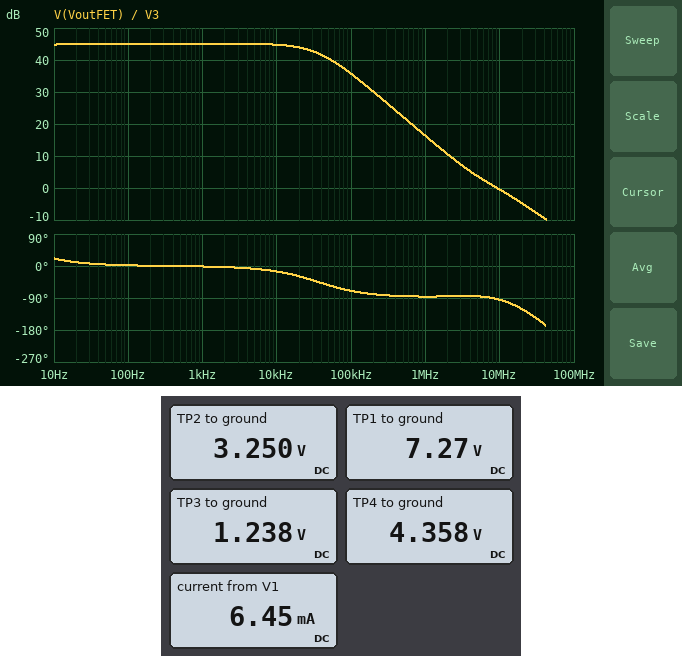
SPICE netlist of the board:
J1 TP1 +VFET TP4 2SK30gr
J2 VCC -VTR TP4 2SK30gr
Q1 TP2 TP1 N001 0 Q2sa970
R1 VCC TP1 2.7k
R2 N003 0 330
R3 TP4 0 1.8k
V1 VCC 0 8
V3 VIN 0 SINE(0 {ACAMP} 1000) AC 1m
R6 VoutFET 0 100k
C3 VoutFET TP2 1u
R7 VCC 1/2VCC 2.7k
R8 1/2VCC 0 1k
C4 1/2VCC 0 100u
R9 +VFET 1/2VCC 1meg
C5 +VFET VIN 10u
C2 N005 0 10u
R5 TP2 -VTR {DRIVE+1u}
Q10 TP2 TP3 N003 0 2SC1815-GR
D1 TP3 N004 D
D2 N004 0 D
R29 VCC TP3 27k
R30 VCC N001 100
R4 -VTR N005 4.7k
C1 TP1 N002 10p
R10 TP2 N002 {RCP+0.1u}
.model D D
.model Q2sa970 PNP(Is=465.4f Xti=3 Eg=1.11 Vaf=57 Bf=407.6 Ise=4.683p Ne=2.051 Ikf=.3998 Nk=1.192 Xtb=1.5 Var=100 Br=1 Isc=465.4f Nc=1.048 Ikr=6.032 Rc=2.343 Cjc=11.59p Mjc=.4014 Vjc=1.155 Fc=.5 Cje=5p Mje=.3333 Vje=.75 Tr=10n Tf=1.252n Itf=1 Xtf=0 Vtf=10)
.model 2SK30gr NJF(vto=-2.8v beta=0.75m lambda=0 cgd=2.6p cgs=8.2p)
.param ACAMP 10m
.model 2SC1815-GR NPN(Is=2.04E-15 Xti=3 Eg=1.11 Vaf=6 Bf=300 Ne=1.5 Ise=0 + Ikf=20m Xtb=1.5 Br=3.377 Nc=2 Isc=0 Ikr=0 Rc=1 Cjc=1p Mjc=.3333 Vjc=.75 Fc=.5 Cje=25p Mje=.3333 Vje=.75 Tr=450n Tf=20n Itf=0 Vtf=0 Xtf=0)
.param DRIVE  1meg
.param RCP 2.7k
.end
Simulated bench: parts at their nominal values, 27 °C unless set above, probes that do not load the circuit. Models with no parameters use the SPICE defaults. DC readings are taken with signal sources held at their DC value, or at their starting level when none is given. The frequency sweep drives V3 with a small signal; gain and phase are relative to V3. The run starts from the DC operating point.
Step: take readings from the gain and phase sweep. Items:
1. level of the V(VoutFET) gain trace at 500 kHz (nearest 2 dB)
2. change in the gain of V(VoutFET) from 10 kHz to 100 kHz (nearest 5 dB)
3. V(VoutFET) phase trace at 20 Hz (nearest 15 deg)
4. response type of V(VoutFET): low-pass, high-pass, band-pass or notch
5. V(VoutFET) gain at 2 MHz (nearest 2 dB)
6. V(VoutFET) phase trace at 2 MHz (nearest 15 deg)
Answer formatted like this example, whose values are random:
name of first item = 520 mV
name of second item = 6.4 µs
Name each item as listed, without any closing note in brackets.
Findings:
level of the V(VoutFET) gain trace at 500 kHz = 22 dB
change in the gain of V(VoutFET) from 10 kHz to 100 kHz = -10 dB
V(VoutFET) phase trace at 20 Hz = 15 deg
response type of V(VoutFET): low-pass, high-pass, band-pass or notch = low-pass
V(VoutFET) gain at 2 MHz = 10 dB
V(VoutFET) phase trace at 2 MHz = -90 deg
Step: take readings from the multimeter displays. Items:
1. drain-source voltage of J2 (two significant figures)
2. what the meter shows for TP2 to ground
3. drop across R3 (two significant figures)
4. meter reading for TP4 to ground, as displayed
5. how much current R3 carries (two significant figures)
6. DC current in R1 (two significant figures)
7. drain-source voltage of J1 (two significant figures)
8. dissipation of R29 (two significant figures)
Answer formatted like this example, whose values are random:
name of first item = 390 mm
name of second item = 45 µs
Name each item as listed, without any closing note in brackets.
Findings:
drain-source voltage of J2 = 3.6 V
what the meter shows for TP2 to ground = 3.250 V
drop across R3 = 4.4 V
meter reading for TP4 to ground, as displayed = 4.358 V
how much current R3 carries = 2.4 mA
DC current in R1 = 270 µA
drain-source voltage of J1 = 2.9 V
dissipation of R29 = 1.7 mW
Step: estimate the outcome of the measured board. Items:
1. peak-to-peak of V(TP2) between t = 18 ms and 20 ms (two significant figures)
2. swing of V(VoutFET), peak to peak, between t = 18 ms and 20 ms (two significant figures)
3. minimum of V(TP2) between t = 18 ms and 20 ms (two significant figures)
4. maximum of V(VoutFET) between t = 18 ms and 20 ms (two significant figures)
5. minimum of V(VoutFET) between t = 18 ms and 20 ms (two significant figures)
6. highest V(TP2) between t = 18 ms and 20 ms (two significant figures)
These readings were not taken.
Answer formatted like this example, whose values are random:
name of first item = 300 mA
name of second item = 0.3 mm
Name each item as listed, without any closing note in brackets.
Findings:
peak-to-peak of V(TP2) between t = 18 ms and 20 ms = 3.6 V
swing of V(VoutFET), peak to peak, between t = 18 ms and 20 ms = 3.6 V
minimum of V(TP2) between t = 18 ms and 20 ms = 1.5 V
maximum of V(VoutFET) between t = 18 ms and 20 ms = 1.8 V
minimum of V(VoutFET) between t = 18 ms and 20 ms = -1.8 V
highest V(TP2) between t = 18 ms and 20 ms = 5.1 V
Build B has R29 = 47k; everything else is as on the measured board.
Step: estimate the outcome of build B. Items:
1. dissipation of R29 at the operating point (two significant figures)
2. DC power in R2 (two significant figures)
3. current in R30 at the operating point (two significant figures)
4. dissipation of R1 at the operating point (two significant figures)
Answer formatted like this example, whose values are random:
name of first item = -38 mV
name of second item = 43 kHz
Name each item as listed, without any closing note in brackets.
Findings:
dissipation of R29 at the operating point = 980 µW
DC power in R2 = 780 µW
current in R30 at the operating point = 1.5 mA
dissipation of R1 at the operating point = 190 µW
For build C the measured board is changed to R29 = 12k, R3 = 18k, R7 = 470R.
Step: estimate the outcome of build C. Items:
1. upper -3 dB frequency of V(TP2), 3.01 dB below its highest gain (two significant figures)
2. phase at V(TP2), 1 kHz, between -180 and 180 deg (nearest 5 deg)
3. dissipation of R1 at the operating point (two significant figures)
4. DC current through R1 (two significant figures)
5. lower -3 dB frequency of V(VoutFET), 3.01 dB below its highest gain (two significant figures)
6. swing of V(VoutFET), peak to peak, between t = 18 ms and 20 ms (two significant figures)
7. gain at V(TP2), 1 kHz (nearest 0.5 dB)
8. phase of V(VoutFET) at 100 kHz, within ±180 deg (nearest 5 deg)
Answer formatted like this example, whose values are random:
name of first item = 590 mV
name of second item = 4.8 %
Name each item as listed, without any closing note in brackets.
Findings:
upper -3 dB frequency of V(TP2), 3.01 dB below its highest gain = 35 kHz
phase at V(TP2), 1 kHz, between -180 and 180 deg = 0 deg
dissipation of R1 at the operating point = 210 µW
DC current through R1 = 280 µA
lower -3 dB frequency of V(VoutFET), 3.01 dB below its highest gain = 2.1 Hz
swing of V(VoutFET), peak to peak, between t = 18 ms and 20 ms = 330 mV
gain at V(TP2), 1 kHz = 24.5 dB
phase of V(VoutFET) at 100 kHz, within ±180 deg = -75 deg
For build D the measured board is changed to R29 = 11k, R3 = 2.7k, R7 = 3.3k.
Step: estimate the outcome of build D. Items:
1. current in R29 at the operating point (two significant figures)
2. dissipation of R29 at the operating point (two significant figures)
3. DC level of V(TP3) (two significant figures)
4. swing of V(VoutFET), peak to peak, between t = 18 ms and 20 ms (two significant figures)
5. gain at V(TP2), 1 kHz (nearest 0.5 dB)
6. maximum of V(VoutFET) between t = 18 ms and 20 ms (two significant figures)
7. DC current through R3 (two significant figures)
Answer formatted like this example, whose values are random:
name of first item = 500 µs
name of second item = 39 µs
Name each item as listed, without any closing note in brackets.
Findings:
current in R29 at the operating point = 610 µA
dissipation of R29 at the operating point = 4.1 mW
DC level of V(TP3) = 1.3 V
swing of V(VoutFET), peak to peak, between t = 18 ms and 20 ms = 3.4 V
gain at V(TP2), 1 kHz = 44.5 dB
maximum of V(VoutFET) between t = 18 ms and 20 ms = 1.7 V
DC current through R3 = 1.5 mA
